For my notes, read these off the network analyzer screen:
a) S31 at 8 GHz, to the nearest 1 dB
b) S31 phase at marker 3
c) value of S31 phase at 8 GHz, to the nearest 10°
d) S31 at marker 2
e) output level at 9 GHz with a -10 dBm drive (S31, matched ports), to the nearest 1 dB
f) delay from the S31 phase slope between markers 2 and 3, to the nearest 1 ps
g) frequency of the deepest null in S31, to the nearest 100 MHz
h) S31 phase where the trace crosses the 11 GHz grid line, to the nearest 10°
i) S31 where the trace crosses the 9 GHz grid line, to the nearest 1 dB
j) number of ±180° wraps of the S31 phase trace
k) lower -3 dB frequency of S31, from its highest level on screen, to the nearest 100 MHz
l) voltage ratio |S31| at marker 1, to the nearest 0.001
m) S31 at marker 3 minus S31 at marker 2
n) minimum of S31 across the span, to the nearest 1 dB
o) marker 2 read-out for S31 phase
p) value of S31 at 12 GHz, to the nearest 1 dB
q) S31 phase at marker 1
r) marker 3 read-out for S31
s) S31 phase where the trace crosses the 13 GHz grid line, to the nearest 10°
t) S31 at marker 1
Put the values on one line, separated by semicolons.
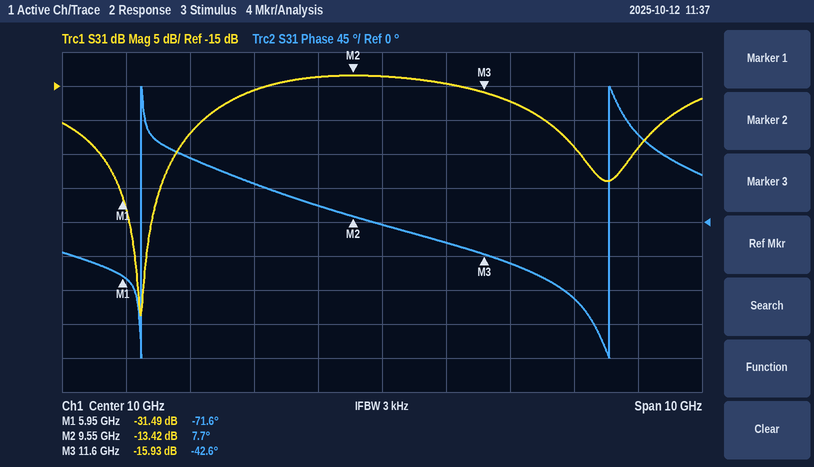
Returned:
-16 dB; -42.6°; 50°; -13.42 dB; -24 dBm; 68 ps; 6.2 GHz; -30°; -14 dB; 2; 7.8 GHz; 0.027; -2.51 dB; -49 dB; 7.7°; -17 dB; -71.6°; -15.93 dB; -100°; -31.49 dB
